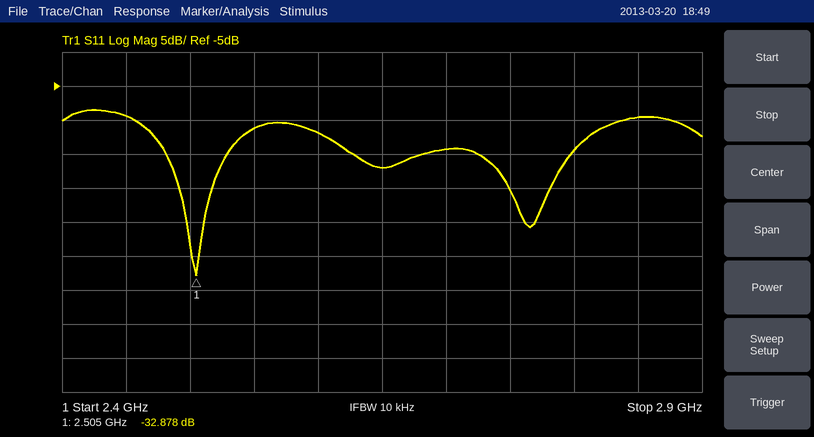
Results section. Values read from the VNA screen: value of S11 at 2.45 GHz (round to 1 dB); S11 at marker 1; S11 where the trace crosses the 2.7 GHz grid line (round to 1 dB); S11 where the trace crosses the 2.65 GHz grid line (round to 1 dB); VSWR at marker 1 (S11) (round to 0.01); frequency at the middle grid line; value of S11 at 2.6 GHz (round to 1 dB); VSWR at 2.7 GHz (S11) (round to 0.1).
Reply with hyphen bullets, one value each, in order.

- -9 dB
- -32.878 dB
- -14 dB
- -17 dB
- 1.05
- 2.65 GHz
- -12 dB
- 1.5
